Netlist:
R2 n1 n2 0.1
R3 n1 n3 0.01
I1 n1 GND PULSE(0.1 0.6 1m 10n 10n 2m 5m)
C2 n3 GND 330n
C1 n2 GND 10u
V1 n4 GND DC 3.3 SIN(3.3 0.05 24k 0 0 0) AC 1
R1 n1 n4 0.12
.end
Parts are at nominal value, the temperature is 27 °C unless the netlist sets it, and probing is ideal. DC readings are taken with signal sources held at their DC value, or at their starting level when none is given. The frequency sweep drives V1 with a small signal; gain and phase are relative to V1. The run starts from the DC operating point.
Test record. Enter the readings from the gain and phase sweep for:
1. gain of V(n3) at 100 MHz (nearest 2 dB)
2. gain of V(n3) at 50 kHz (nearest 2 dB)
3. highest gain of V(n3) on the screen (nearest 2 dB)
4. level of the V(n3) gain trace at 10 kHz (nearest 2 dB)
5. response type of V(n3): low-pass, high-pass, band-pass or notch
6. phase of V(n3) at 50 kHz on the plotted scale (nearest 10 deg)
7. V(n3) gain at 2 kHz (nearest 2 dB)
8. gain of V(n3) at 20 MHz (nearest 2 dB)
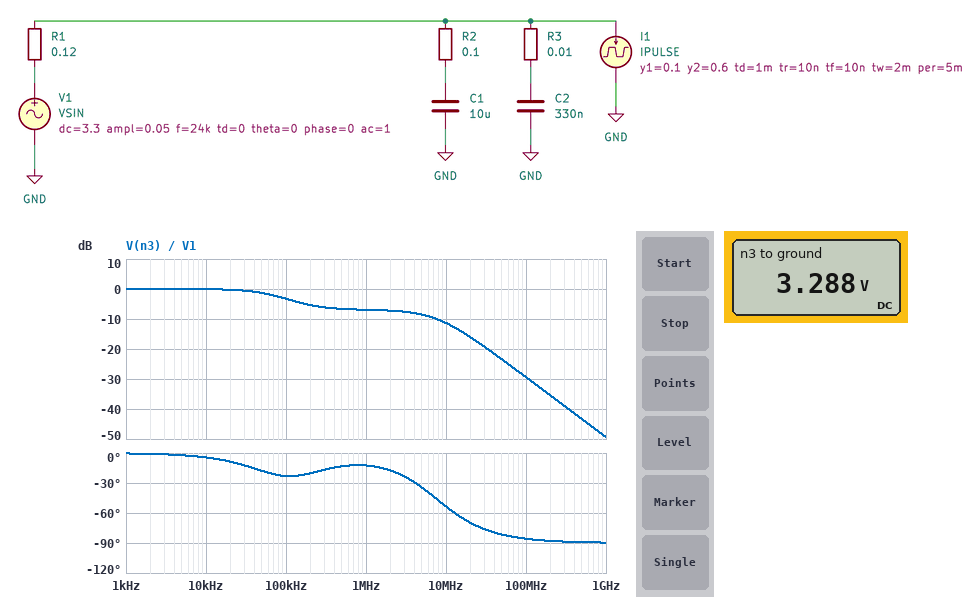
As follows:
-30 dB
-2 dB
0 dB
0 dB
low-pass
-20 deg
0 dB
-16 dB
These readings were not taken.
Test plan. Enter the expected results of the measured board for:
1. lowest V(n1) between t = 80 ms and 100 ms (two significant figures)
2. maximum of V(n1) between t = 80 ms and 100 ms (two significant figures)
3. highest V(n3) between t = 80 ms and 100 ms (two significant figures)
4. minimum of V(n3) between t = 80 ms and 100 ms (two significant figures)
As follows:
3.2 V
3.3 V
3.3 V
3.2 V
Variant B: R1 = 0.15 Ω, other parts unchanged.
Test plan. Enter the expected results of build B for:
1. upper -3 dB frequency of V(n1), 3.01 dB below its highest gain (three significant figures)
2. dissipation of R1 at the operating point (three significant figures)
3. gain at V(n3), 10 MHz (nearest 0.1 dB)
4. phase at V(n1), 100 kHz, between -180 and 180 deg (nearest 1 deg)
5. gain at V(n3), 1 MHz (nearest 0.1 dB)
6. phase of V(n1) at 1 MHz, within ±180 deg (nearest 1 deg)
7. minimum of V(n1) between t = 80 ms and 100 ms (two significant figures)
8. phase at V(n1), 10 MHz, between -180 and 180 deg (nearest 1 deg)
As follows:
75.9 kHz
1.50 mW
-12.9 dB
-26 deg
-8.1 dB
-12 deg
3.2 V
-44 deg
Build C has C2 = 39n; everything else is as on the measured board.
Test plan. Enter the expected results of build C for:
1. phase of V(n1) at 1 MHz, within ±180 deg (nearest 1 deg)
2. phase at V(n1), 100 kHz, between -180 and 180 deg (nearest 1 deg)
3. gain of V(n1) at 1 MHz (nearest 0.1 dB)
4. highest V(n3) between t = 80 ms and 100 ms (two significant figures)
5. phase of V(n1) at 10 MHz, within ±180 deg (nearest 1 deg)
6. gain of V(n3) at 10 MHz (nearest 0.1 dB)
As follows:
-6 deg
-22 deg
-6.8 dB
3.3 V
-8 deg
-7.0 dB
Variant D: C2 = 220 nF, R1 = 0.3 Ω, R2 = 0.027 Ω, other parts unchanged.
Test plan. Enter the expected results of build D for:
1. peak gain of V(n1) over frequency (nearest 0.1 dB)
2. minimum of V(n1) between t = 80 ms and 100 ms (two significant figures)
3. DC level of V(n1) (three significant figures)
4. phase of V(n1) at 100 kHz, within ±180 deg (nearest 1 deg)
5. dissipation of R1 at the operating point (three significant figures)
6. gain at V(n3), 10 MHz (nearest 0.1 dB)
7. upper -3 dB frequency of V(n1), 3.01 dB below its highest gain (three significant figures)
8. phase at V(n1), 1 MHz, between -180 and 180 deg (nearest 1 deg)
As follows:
0 dB
3.1 V
3.27 V
-55 deg
3.00 mW
-22.7 dB
48.1 kHz
-30 deg
